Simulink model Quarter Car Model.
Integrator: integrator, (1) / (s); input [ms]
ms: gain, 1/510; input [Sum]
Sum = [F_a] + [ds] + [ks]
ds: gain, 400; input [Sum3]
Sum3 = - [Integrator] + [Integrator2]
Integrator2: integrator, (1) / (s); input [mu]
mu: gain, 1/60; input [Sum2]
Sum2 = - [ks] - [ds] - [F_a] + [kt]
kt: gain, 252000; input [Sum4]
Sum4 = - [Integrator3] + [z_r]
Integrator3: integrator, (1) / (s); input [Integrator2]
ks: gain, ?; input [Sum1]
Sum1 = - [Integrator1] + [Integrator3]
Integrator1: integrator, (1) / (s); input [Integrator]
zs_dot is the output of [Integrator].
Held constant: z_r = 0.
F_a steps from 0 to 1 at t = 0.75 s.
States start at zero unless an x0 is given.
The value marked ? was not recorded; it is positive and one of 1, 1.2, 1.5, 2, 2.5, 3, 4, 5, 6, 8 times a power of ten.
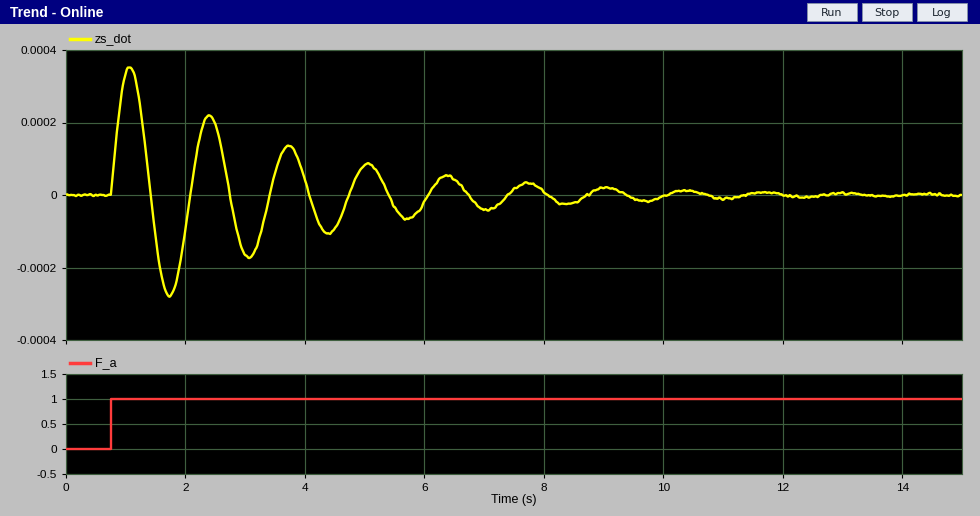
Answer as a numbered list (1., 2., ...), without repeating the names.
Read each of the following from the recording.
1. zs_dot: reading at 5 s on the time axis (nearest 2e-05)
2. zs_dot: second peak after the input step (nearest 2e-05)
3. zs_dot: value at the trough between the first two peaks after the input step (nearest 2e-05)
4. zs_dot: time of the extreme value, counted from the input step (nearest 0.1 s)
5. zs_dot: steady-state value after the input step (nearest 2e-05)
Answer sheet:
1. 0.00008
2. 0.00022
3. -0.00028
4. 0.3 s
5. 0.00000
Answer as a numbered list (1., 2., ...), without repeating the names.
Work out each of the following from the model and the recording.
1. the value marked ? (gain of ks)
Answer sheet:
1. 12000
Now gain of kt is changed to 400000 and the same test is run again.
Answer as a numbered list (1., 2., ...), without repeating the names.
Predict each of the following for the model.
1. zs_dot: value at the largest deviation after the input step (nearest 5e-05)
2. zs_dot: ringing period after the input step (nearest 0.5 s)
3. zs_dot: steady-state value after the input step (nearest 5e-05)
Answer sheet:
1. 0.00035
2. 1.5 s
3. 0.00000
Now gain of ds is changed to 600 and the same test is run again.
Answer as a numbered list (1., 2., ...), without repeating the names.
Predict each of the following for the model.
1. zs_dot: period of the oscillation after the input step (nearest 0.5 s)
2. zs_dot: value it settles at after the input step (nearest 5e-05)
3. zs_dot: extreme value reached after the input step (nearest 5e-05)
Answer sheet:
1. 1.5 s
2. 0.00000
3. 0.00035
